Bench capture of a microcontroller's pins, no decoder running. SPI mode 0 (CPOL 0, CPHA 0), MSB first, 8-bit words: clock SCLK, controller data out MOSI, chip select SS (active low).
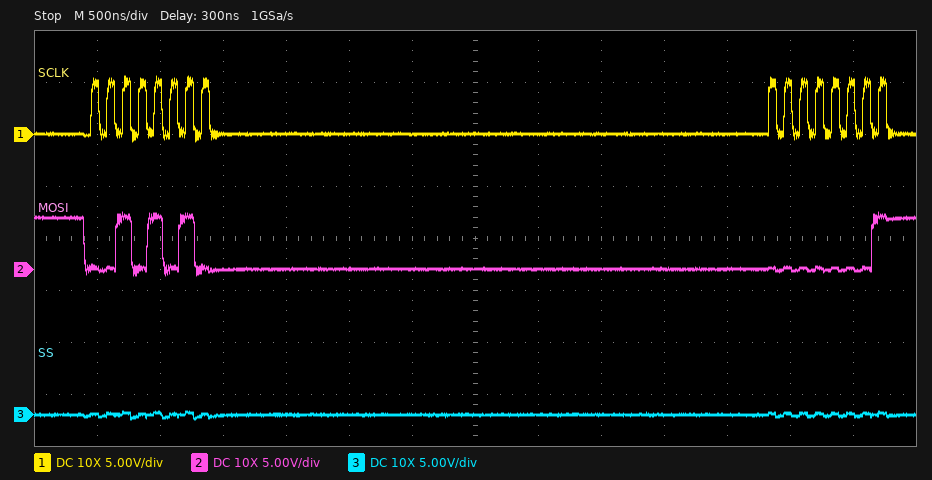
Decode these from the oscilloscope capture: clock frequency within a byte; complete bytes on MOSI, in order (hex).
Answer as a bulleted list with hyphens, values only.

- 8 MHz
- 2A 01
